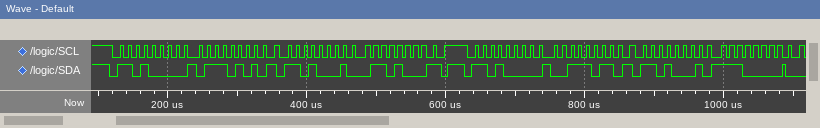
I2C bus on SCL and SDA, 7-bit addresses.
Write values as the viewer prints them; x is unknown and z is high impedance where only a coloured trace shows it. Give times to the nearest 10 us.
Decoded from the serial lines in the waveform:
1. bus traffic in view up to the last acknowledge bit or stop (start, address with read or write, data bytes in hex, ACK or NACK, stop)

start, address 68 write ACK, 75 ACK, repeated start, address 68 read ACK, 68 NACK, stop, start, address 68 write ACK, 3B ACK, repeated start, address 68 read ACK, E0 ACK
